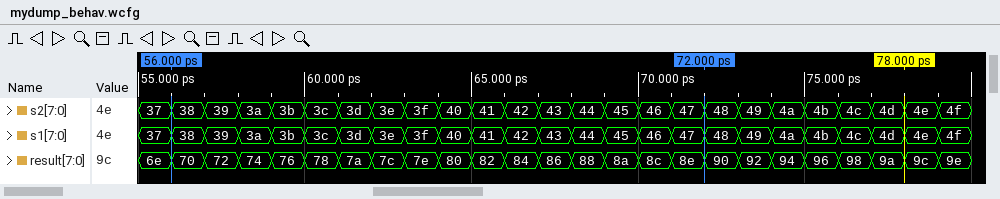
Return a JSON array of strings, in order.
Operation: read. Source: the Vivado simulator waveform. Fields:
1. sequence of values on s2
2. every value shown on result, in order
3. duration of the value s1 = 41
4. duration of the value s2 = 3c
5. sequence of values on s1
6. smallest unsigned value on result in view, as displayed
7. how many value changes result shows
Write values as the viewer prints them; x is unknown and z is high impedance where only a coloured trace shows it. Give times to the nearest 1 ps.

["37, 38, 39, 3a, 3b, 3c, 3d, 3e, 3f, 40, 41, 42, 43, 44, 45, 46, 47, 48, 49, 4a, 4b, 4c, 4d, 4e, 4f", "6e, 70, 72, 74, 76, 78, 7a, 7c, 7e, 80, 82, 84, 86, 88, 8a, 8c, 8e, 90, 92, 94, 96, 98, 9a, 9c, 9e", "1 ps", "1 ps", "37, 38, 39, 3a, 3b, 3c, 3d, 3e, 3f, 40, 41, 42, 43, 44, 45, 46, 47, 48, 49, 4a, 4b, 4c, 4d, 4e, 4f", "6e", "24"]
